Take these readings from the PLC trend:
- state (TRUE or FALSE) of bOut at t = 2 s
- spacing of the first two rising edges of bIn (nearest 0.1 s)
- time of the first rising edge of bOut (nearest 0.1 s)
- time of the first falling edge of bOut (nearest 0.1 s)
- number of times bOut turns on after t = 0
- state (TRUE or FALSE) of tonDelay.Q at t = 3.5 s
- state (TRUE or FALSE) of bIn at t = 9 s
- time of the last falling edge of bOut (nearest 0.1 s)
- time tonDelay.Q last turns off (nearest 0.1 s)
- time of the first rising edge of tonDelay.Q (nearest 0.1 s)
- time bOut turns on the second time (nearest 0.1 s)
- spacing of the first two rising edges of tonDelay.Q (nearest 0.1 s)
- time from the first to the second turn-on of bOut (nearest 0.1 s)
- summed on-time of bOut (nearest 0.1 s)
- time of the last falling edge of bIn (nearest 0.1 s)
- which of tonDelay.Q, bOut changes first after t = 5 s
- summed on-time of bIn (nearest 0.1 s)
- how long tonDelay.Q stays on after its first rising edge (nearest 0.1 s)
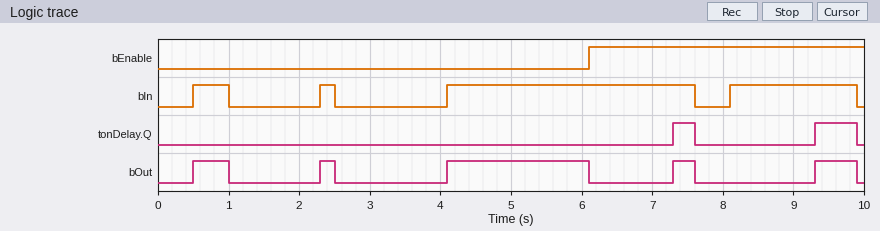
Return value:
FALSE
1.8 s
0.5 s
1.0 s
5
FALSE
TRUE
9.9 s
9.9 s
7.3 s
2.3 s
2.0 s
1.8 s
3.6 s
9.9 s
bOut
6.0 s
0.3 s
